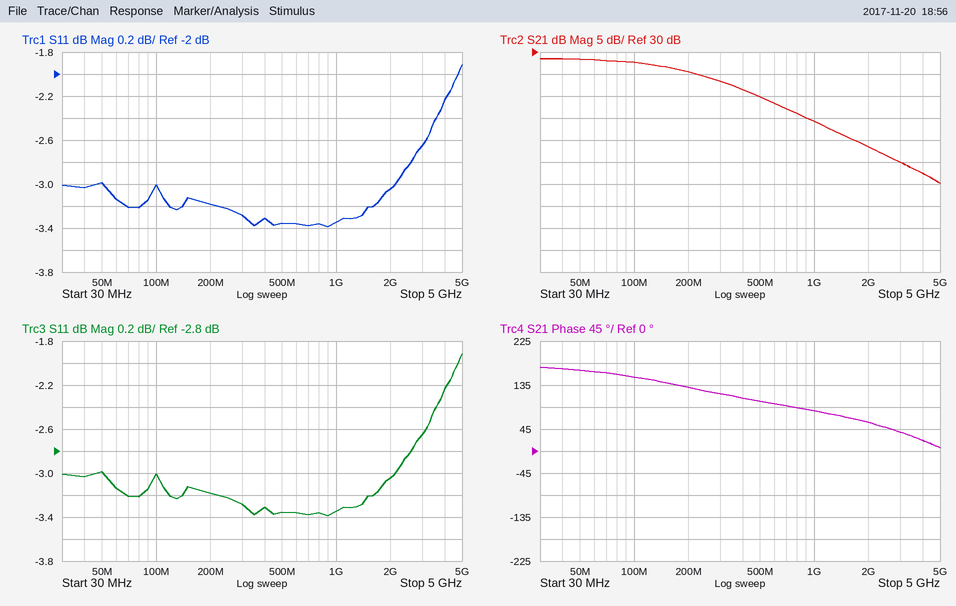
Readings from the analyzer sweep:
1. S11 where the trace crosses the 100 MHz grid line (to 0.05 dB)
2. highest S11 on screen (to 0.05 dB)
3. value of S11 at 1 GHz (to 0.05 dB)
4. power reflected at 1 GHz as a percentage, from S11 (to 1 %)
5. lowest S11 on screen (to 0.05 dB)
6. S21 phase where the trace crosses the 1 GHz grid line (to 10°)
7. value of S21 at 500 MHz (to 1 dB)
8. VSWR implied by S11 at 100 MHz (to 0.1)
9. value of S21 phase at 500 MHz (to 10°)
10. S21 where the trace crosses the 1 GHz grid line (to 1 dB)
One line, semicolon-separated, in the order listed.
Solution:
-3.00 dB; -1.90 dB; -3.35 dB; 46 %; -3.40 dB; 80°; 20 dB; 5.8; 100°; 14 dB
